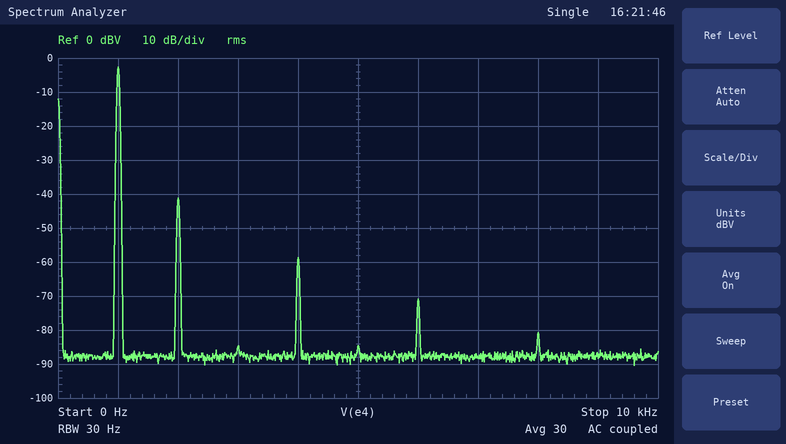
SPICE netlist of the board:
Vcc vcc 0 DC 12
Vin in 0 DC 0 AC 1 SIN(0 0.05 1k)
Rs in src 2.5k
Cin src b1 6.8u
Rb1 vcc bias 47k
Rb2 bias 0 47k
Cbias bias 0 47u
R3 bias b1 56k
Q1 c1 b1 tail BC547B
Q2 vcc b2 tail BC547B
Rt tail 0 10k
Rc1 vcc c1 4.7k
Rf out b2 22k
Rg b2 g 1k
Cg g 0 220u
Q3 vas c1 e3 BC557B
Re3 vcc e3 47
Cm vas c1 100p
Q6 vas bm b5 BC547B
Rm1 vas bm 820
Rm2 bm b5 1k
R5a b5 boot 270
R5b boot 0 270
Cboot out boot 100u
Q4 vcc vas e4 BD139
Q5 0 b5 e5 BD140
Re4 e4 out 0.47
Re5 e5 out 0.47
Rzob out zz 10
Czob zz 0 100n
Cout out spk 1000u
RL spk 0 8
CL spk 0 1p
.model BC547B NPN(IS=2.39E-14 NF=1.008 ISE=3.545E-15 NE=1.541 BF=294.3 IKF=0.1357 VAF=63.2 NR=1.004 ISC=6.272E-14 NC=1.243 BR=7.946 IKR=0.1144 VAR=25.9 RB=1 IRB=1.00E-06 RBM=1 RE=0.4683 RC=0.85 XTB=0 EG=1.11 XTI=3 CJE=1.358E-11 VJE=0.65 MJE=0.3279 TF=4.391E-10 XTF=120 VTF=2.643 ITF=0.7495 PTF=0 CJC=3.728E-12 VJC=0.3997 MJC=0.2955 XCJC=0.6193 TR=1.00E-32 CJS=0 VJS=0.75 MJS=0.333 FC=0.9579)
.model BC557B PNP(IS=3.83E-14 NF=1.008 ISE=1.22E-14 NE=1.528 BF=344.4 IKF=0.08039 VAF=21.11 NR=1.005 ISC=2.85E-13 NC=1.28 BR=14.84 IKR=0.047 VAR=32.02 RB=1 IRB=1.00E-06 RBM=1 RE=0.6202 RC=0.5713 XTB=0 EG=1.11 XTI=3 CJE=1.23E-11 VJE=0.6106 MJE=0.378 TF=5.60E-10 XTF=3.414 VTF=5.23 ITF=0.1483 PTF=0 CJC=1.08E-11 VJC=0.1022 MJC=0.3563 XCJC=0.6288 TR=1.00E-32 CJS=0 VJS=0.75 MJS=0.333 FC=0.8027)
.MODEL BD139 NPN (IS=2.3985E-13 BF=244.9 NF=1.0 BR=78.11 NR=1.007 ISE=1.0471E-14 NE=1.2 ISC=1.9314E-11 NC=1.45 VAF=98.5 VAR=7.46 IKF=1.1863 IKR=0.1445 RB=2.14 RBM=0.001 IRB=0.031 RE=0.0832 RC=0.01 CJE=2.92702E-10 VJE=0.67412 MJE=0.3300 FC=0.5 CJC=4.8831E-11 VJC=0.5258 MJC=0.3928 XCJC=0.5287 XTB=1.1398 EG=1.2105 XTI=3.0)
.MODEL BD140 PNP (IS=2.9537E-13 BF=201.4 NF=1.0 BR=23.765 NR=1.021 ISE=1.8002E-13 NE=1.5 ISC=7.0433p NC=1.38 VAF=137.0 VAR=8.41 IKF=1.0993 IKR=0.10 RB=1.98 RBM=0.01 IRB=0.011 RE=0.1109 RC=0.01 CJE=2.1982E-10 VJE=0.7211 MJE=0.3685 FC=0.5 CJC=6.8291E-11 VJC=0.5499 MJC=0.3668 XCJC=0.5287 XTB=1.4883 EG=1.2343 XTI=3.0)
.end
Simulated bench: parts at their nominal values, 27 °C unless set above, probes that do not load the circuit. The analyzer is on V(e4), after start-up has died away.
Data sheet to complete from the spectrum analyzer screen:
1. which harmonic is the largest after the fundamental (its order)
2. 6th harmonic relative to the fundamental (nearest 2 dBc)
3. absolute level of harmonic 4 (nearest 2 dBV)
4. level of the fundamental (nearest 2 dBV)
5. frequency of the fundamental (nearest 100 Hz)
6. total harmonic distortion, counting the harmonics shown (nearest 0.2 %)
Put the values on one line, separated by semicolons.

2; -68 dBc; -58 dBV; -2 dBV; 1.0 kHz; 1.2 %
